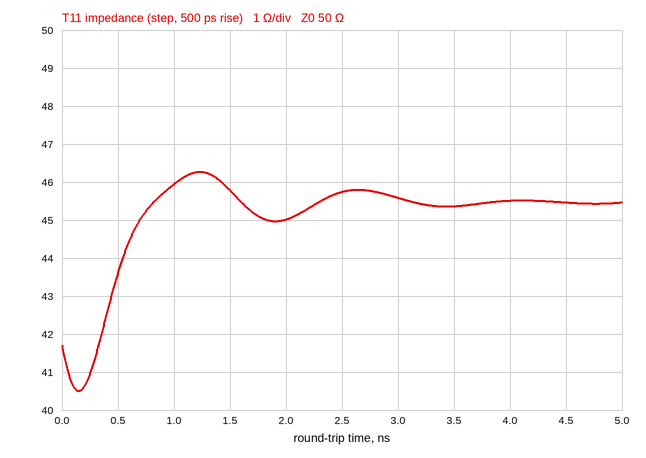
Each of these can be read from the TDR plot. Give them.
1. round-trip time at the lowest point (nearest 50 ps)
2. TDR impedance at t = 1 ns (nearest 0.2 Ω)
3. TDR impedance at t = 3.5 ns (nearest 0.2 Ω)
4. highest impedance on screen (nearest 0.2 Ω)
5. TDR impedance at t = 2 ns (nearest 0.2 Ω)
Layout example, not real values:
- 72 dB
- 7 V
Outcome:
- 150 ps
- 46.0 Ω
- 45.4 Ω
- 46.2 Ω
- 45.0 Ω
